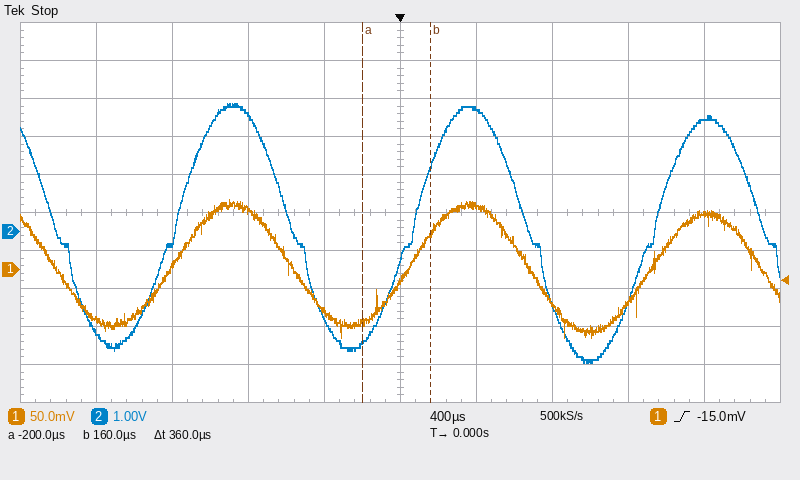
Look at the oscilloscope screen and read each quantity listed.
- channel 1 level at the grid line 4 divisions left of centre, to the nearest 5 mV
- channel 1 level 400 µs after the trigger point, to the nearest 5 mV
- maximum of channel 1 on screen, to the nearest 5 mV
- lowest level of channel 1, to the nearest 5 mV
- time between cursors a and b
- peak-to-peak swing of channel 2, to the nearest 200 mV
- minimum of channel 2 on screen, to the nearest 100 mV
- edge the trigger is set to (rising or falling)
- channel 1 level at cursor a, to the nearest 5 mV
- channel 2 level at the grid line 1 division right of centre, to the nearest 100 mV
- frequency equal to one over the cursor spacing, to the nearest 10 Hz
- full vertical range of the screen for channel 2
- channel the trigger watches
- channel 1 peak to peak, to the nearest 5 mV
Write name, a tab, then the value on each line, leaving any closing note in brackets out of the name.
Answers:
channel 1 level at the grid line 4 divisions left of centre, to the nearest 5 mV	-65 mV
channel 1 level 400 µs after the trigger point, to the nearest 5 mV	85 mV
maximum of channel 1 on screen, to the nearest 5 mV	90 mV
lowest level of channel 1, to the nearest 5 mV	-90 mV
time between cursors a and b	360 µs
peak-to-peak swing of channel 2, to the nearest 200 mV	6.8 V
minimum of channel 2 on screen, to the nearest 100 mV	-3.4 V
edge the trigger is set to	rising
channel 1 level at cursor a, to the nearest 5 mV	-70 mV
channel 2 level at the grid line 1 division right of centre, to the nearest 100 mV	3.2 V
frequency equal to one over the cursor spacing, to the nearest 10 Hz	2.78 kHz
full vertical range of the screen for channel 2	10 V
channel the trigger watches	channel 1
channel 1 peak to peak, to the nearest 5 mV	180 mV
